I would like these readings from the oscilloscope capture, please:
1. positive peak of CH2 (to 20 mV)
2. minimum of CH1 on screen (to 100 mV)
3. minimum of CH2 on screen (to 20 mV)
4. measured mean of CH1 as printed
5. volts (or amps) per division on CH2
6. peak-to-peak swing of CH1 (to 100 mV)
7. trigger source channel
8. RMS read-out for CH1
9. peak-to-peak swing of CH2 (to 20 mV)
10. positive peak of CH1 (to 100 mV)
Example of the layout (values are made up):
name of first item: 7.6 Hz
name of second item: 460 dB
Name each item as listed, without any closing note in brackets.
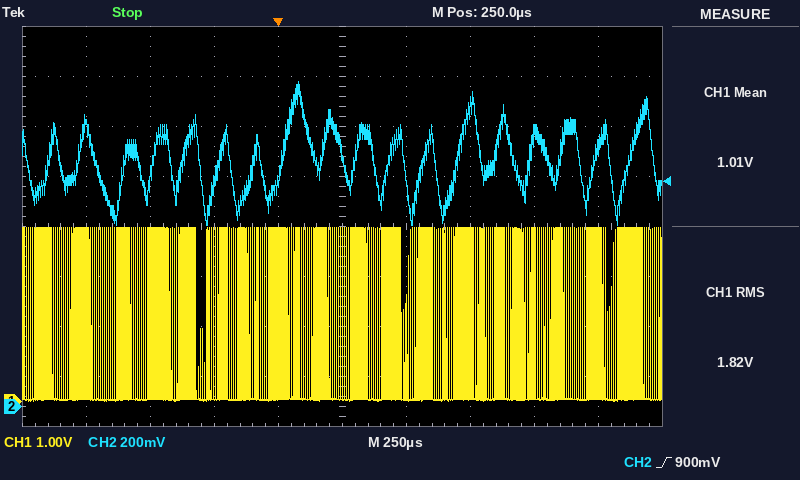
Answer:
positive peak of CH2: 1.30 V
minimum of CH1 on screen: 0.0 V
minimum of CH2 on screen: 720 mV
measured mean of CH1 as printed: 1.01 V
volts (or amps) per division on CH2: 200 mV
peak-to-peak swing of CH1: 3.5 V
trigger source channel: CH2
RMS read-out for CH1: 1.82 V
peak-to-peak swing of CH2: 580 mV
positive peak of CH1: 3.5 V
